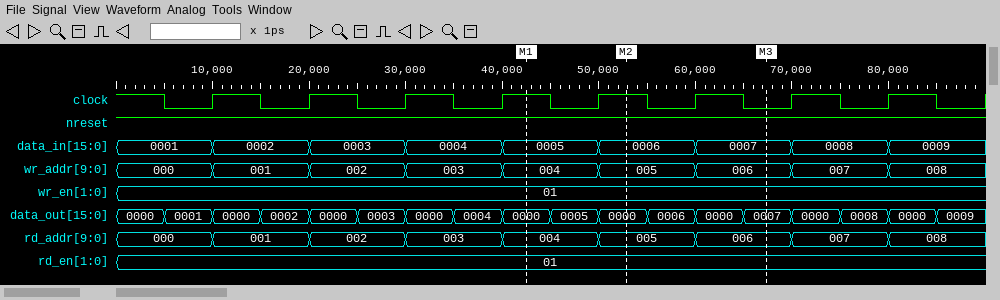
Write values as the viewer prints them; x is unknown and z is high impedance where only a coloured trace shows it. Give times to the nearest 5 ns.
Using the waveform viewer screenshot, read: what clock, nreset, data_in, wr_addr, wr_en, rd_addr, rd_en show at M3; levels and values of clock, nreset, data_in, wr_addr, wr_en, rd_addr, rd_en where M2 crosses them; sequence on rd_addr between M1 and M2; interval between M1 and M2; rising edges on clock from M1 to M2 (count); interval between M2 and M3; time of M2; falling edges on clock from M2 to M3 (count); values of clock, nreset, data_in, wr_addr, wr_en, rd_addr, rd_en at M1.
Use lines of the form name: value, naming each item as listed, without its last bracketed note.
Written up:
what clock, nreset, data_in, wr_addr, wr_en, rd_addr, rd_en show at M3: clock=0, nreset=1, data_in=0007, wr_addr=006, wr_en=01, rd_addr=006, rd_en=01
levels and values of clock, nreset, data_in, wr_addr, wr_en, rd_addr, rd_en where M2 crosses them: clock=1, nreset=1, data_in=0006, wr_addr=005, wr_en=01, rd_addr=005, rd_en=01
sequence on rd_addr between M1 and M2: 004, 005
interval between M1 and M2: 10 ns
rising edges on clock from M1 to M2: 1
interval between M2 and M3: 15 ns
time of M2: 55 ns
falling edges on clock from M2 to M3: 2
values of clock, nreset, data_in, wr_addr, wr_en, rd_addr, rd_en at M1: clock=1, nreset=1, data_in=0005, wr_addr=004, wr_en=01, rd_addr=004, rd_en=01
